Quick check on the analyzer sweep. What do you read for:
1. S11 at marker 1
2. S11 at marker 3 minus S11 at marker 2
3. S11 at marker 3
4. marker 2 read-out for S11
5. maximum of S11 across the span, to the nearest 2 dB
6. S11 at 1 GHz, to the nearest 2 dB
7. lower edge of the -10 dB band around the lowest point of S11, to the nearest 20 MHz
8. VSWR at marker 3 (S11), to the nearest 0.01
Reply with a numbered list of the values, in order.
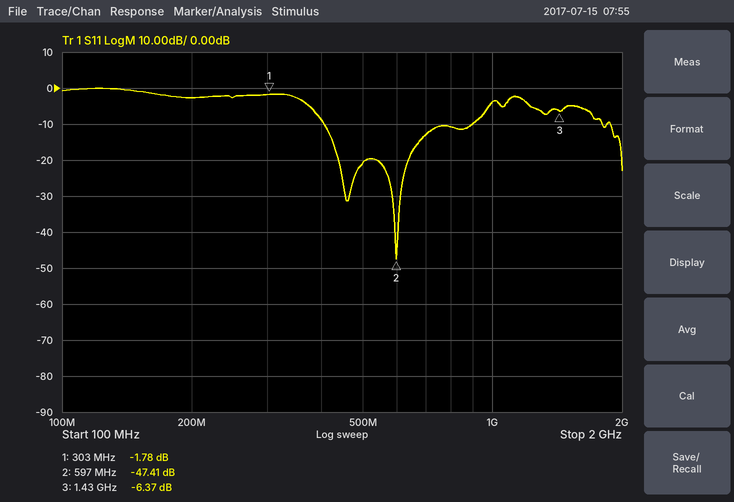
1. -1.78 dB
2. 41.04 dB
3. -6.37 dB
4. -47.41 dB
5. 0 dB
6. -4 dB
7. 400 MHz
8. 2.85
